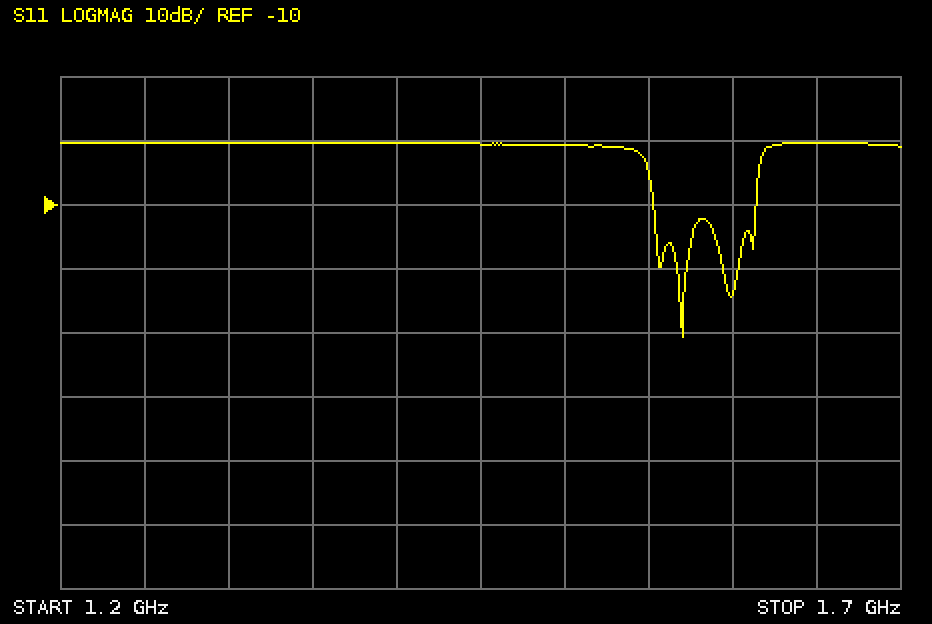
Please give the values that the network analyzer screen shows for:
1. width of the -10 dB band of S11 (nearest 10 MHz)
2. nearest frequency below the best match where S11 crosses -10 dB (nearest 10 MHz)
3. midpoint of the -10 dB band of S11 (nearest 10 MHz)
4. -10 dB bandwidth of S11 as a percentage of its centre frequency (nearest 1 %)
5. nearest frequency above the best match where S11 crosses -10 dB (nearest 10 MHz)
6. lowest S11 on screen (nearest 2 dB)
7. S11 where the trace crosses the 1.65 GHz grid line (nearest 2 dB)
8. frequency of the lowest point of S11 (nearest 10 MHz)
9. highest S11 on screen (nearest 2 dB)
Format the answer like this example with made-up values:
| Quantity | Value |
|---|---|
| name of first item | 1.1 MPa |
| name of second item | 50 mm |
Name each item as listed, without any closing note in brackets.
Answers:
| Quantity | Value |
|---|---|
| width of the -10 dB band of S11 | 60 MHz |
| nearest frequency below the best match where S11 crosses -10 dB | 1.55 GHz |
| midpoint of the -10 dB band of S11 | 1.58 GHz |
| -10 dB bandwidth of S11 as a percentage of its centre frequency | 4 % |
| nearest frequency above the best match where S11 crosses -10 dB | 1.61 GHz |
| lowest S11 on screen | -30 dB |
| S11 where the trace crosses the 1.65 GHz grid line | 0 dB |
| frequency of the lowest point of S11 | 1.57 GHz |
| highest S11 on screen | 0 dB |
